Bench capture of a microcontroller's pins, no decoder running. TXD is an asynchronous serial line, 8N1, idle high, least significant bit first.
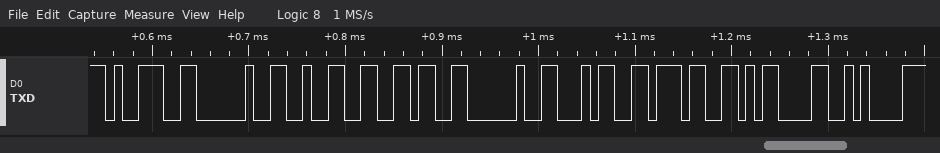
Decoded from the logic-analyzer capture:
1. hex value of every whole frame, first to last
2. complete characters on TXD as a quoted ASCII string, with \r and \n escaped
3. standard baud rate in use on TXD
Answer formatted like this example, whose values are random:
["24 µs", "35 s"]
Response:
["0x39 0x20 0x32 0x36 0x20 0x34 0x37 0x0D 0x0A", "\"9 26 47\\r\\n\"", "115200 baud"]
